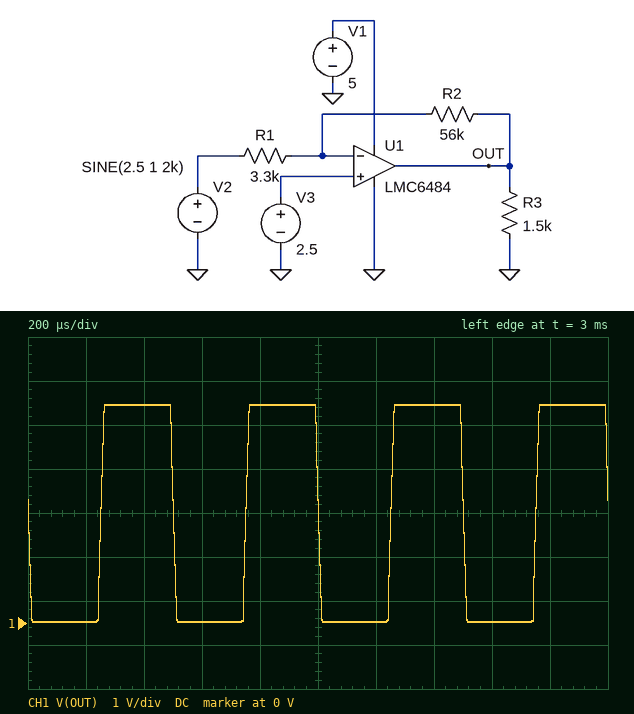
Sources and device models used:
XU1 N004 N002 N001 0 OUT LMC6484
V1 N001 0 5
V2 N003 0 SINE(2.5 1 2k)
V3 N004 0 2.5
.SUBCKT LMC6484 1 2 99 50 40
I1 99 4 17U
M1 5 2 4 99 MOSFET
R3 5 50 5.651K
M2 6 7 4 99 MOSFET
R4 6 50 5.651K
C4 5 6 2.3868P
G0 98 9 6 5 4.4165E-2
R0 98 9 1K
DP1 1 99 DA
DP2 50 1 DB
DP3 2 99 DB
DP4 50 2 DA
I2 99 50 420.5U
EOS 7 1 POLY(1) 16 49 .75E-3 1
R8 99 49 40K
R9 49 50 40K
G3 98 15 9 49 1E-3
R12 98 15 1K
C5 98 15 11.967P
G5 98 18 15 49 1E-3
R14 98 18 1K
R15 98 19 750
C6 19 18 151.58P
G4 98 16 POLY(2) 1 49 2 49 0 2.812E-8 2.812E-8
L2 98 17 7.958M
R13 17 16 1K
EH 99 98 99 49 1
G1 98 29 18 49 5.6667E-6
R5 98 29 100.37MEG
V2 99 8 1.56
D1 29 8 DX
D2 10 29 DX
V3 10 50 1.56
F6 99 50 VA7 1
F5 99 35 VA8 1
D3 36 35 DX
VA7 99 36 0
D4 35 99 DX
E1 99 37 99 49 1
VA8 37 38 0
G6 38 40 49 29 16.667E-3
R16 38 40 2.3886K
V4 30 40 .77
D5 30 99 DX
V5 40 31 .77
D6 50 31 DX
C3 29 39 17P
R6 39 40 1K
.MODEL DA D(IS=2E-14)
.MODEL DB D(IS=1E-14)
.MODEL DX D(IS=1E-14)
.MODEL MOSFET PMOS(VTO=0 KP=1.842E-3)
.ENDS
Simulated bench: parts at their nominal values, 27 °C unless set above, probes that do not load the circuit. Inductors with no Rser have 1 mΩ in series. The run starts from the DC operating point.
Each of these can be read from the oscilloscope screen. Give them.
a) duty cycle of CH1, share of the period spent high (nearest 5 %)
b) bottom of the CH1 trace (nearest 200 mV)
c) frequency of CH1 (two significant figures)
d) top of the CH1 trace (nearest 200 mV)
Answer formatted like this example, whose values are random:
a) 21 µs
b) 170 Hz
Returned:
a) 50 %
b) 0 V
c) 2.0 kHz
d) 5.0 V
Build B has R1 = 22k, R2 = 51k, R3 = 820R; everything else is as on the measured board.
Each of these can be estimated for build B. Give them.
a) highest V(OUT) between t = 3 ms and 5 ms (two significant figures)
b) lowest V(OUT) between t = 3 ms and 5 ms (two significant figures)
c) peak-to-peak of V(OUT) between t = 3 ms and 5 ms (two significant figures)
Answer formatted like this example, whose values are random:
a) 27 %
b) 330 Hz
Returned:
a) 4.8 V
b) 180 mV
c) 4.6 V
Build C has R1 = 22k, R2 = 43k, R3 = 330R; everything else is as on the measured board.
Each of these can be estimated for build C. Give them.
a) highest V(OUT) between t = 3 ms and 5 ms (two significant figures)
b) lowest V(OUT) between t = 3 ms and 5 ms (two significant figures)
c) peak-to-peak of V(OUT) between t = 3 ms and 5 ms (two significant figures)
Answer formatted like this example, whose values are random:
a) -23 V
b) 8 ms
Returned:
a) 4.5 V
b) 550 mV
c) 3.9 V
